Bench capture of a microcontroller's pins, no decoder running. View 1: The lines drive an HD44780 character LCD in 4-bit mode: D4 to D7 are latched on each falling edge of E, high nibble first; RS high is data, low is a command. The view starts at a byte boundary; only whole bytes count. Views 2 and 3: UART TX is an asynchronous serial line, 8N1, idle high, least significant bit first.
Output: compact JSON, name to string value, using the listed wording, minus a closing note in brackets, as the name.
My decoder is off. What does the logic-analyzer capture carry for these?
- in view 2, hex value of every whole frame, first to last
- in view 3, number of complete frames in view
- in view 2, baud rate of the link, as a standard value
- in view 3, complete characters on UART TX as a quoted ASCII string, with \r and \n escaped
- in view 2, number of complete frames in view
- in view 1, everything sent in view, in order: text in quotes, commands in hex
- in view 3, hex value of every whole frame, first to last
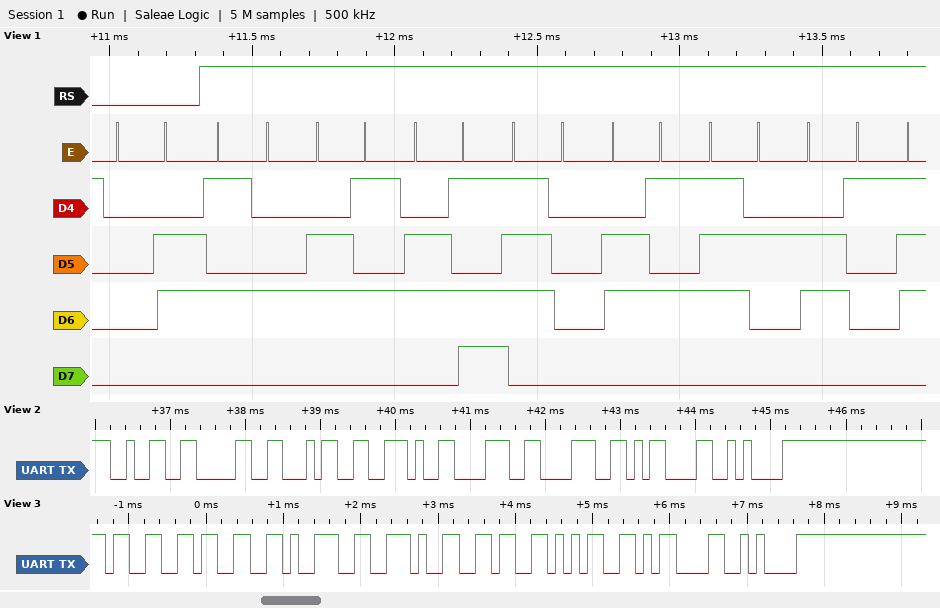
{"in view 2, hex value of every whole frame, first to last": "32 30 34 2E 38 38 0D 0A", "in view 3, number of complete frames in view": "8", "in view 2, baud rate of the link, as a standard value": "9600 baud", "in view 3, complete characters on UART TX as a quoted ASCII string, with \\r and \\n escaped": "\"339.65\\r\\n\"", "in view 2, number of complete frames in view": "8", "in view 1, everything sent in view, in order: text in quotes, commands in hex": "0x06 \"Tempera\"", "in view 3, hex value of every whole frame, first to last": "33 33 39 2E 36 35 0D 0A"}
